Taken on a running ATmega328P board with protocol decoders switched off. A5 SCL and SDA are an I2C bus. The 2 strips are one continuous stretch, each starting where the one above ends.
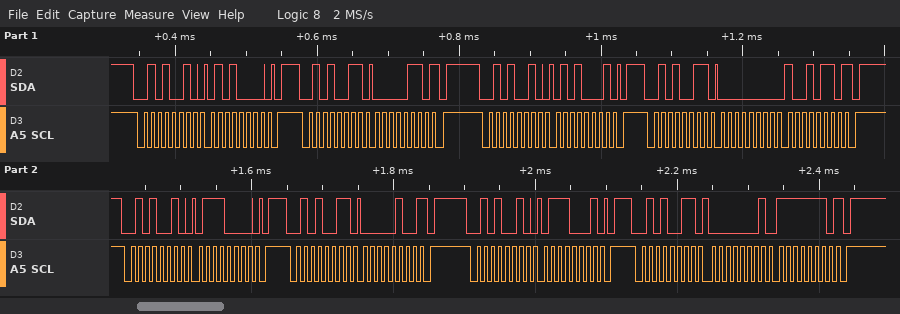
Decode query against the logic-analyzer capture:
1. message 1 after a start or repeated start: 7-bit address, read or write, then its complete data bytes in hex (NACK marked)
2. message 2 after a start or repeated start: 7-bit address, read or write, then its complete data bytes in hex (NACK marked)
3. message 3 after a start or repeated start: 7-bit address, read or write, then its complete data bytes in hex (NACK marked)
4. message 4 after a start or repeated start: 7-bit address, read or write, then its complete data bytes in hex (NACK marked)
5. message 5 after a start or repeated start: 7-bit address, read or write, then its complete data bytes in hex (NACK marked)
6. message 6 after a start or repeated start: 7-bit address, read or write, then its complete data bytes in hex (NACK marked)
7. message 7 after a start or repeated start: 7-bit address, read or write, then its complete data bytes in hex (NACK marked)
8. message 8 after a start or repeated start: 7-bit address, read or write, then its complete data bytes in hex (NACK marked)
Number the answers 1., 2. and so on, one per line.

1. 0x29 write: 50
2. 0x29 read: 06 NACK
3. 0x29 write: 51
4. 0x29 read: 00 96 NACK
5. 0x29 write: 70
6. 0x29 read: 04 NACK
7. 0x29 write: 71
8. 0x29 read: 01 FE NACK
